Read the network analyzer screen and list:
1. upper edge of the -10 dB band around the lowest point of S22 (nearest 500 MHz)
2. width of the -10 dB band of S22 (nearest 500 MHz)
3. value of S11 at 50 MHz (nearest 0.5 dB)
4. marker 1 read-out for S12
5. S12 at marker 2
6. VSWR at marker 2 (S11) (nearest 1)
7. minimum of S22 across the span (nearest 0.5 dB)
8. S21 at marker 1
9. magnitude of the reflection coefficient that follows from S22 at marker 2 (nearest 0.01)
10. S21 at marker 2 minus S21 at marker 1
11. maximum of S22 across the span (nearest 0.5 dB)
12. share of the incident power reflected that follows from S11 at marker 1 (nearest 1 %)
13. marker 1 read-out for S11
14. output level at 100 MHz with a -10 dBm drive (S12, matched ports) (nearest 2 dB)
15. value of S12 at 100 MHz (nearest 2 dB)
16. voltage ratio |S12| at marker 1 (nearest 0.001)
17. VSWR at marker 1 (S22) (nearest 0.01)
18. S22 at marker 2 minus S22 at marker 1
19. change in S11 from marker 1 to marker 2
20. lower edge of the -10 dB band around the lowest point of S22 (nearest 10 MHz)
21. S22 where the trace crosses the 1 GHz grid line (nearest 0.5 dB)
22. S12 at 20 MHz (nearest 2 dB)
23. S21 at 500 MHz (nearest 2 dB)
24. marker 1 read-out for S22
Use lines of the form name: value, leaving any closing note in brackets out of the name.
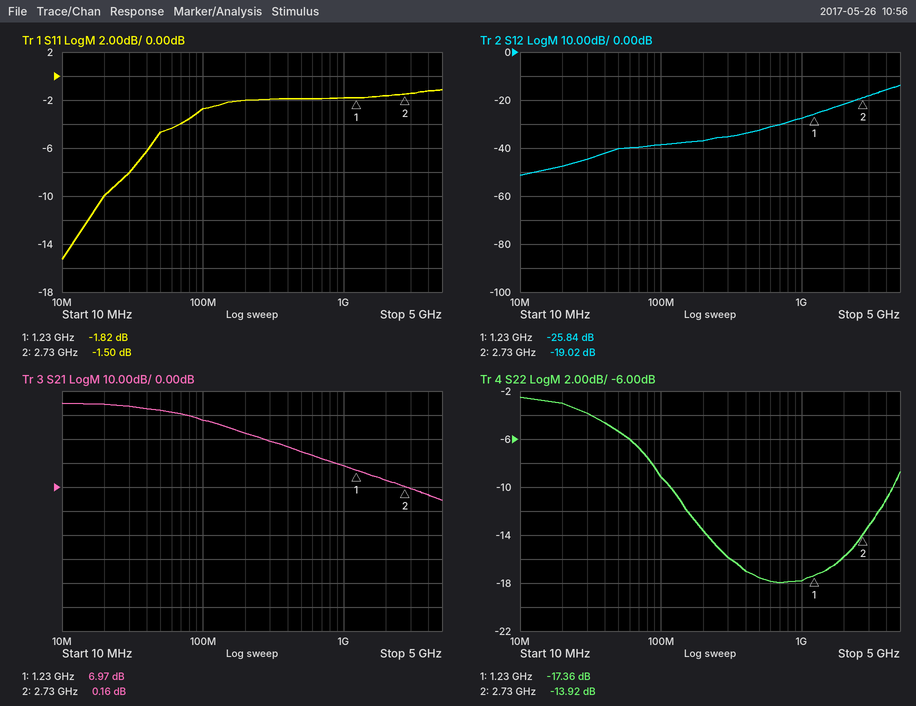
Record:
upper edge of the -10 dB band around the lowest point of S22: 4.5 GHz
width of the -10 dB band of S22: 4.5 GHz
value of S11 at 50 MHz: -4.5 dB
marker 1 read-out for S12: -25.84 dB
S12 at marker 2: -19.02 dB
VSWR at marker 2 (S11): 12
minimum of S22 across the span: -18.0 dB
S21 at marker 1: 6.97 dB
magnitude of the reflection coefficient that follows from S22 at marker 2: 0.20
S21 at marker 2 minus S21 at marker 1: -6.81 dB
maximum of S22 across the span: -2.5 dB
share of the incident power reflected that follows from S11 at marker 1: 66 %
marker 1 read-out for S11: -1.82 dB
output level at 100 MHz with a -10 dBm drive (S12, matched ports): -48 dBm
value of S12 at 100 MHz: -38 dB
voltage ratio |S12| at marker 1: 0.051
VSWR at marker 1 (S22): 1.31
S22 at marker 2 minus S22 at marker 1: 3.44 dB
change in S11 from marker 1 to marker 2: 0.32 dB
lower edge of the -10 dB band around the lowest point of S22: 120 MHz
S22 where the trace crosses the 1 GHz grid line: -18.0 dB
S12 at 20 MHz: -48 dB
S21 at 500 MHz: 14 dB
marker 1 read-out for S22: -17.36 dB
